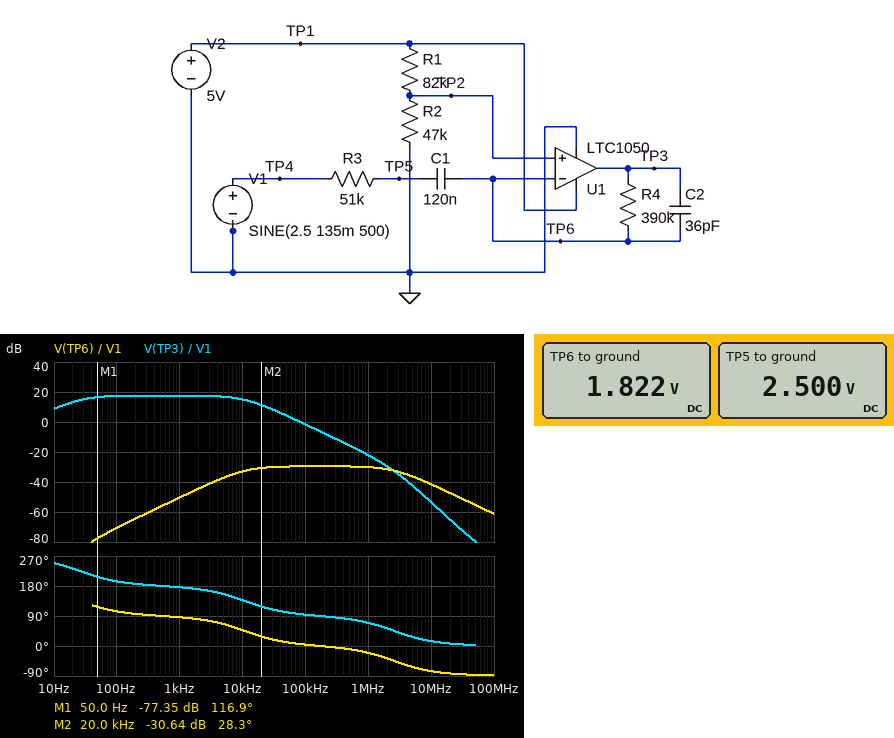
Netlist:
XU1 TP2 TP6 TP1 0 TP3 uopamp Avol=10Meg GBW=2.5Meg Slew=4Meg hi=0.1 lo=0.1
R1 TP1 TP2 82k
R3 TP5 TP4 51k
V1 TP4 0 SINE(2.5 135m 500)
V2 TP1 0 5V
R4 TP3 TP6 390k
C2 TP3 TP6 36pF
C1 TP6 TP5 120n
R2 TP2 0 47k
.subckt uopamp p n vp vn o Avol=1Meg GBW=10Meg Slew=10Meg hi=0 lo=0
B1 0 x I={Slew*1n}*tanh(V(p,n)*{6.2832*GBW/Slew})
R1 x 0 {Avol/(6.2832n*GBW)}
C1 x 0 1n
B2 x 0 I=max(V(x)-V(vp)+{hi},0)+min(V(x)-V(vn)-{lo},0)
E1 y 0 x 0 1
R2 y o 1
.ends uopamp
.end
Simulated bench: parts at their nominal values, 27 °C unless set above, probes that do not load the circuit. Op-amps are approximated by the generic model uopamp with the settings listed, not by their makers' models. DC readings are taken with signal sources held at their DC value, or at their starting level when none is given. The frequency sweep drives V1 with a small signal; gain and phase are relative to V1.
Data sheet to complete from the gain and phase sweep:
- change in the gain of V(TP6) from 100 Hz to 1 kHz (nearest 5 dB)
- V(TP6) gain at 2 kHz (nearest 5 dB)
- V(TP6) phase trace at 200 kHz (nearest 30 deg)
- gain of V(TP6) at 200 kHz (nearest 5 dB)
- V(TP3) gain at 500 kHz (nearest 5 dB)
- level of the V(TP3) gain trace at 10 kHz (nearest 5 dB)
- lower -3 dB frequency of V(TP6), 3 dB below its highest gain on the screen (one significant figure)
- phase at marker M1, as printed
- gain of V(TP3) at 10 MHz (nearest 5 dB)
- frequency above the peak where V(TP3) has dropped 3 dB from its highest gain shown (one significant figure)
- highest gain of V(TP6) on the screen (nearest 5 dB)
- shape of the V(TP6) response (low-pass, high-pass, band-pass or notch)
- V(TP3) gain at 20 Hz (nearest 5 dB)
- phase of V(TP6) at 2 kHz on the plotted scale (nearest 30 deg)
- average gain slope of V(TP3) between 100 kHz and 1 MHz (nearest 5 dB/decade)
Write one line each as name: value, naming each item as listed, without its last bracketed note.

change in the gain of V(TP6) from 100 Hz to 1 kHz: 20 dB
V(TP6) gain at 2 kHz: -45 dB
V(TP6) phase trace at 200 kHz: 0 deg
gain of V(TP6) at 200 kHz: -30 dB
V(TP3) gain at 500 kHz: -15 dB
level of the V(TP3) gain trace at 10 kHz: 15 dB
lower -3 dB frequency of V(TP6), 3 dB below its highest gain on the screen: 10 kHz
phase at marker M1, as printed: 116.9 deg
gain of V(TP3) at 10 MHz: -55 dB
frequency above the peak where V(TP3) has dropped 3 dB from its highest gain shown: 10 kHz
highest gain of V(TP6) on the screen: -30 dB
shape of the V(TP6) response: band-pass
V(TP3) gain at 20 Hz: 15 dB
phase of V(TP6) at 2 kHz on the plotted scale: 90 deg
average gain slope of V(TP3) between 100 kHz and 1 MHz: -20 dB/decade
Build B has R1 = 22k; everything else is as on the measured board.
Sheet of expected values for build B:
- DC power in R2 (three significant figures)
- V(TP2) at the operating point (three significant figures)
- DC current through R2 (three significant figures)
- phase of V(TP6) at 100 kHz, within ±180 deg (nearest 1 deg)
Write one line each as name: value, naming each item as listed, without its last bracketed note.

DC power in R2: 247 µW
V(TP2) at the operating point: 3.41 V
DC current through R2: 72.5 µA
phase of V(TP6) at 100 kHz, within ±180 deg: 4 deg
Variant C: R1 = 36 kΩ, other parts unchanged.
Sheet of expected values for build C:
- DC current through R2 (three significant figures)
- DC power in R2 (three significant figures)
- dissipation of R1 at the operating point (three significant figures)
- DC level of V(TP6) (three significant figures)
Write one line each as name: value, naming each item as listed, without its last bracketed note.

DC current through R2: 60.2 µA
DC power in R2: 171 µW
dissipation of R1 at the operating point: 131 µW
DC level of V(TP6): 2.83 V
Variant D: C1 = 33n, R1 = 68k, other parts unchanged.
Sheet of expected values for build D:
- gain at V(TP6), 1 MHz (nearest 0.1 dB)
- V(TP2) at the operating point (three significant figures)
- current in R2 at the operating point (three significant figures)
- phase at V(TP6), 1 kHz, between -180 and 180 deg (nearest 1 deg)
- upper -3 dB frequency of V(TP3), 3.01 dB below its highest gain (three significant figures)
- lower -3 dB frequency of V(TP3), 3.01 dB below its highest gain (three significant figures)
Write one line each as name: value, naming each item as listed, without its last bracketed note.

gain at V(TP6), 1 MHz: -30.1 dB
V(TP2) at the operating point: 2.04 V
current in R2 at the operating point: 43.5 µA
phase at V(TP6), 1 kHz, between -180 and 180 deg: 90 deg
upper -3 dB frequency of V(TP3), 3.01 dB below its highest gain: 11.1 kHz
lower -3 dB frequency of V(TP3), 3.01 dB below its highest gain: 93.0 Hz
